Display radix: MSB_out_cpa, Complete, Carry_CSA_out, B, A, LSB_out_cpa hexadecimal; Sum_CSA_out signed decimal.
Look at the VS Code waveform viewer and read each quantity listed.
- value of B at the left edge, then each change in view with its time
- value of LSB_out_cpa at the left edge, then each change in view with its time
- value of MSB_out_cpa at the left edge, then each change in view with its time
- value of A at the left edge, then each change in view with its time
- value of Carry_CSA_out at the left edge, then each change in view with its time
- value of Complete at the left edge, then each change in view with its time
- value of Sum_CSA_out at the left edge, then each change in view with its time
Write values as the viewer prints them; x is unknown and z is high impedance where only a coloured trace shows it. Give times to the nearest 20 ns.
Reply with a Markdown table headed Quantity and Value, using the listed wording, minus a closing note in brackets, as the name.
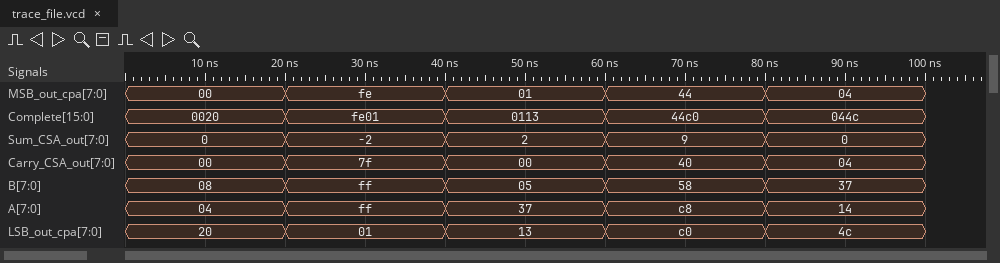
| Quantity | Value |
|---|---|
| value of B at the left edge, then each change in view with its time | 08, ff at 20 ns, 05 at 40 ns, 58 at 60 ns, 37 at 80 ns |
| value of LSB_out_cpa at the left edge, then each change in view with its time | 20, 01 at 20 ns, 13 at 40 ns, c0 at 60 ns, 4c at 80 ns |
| value of MSB_out_cpa at the left edge, then each change in view with its time | 00, fe at 20 ns, 01 at 40 ns, 44 at 60 ns, 04 at 80 ns |
| value of A at the left edge, then each change in view with its time | 04, ff at 20 ns, 37 at 40 ns, c8 at 60 ns, 14 at 80 ns |
| value of Carry_CSA_out at the left edge, then each change in view with its time | 00, 7f at 20 ns, 00 at 40 ns, 40 at 60 ns, 04 at 80 ns |
| value of Complete at the left edge, then each change in view with its time | 0020, fe01 at 20 ns, 0113 at 40 ns, 44c0 at 60 ns, 044c at 80 ns |
| value of Sum_CSA_out at the left edge, then each change in view with its time | 0, -2 at 20 ns, 2 at 40 ns, 9 at 60 ns, 0 at 80 ns |
